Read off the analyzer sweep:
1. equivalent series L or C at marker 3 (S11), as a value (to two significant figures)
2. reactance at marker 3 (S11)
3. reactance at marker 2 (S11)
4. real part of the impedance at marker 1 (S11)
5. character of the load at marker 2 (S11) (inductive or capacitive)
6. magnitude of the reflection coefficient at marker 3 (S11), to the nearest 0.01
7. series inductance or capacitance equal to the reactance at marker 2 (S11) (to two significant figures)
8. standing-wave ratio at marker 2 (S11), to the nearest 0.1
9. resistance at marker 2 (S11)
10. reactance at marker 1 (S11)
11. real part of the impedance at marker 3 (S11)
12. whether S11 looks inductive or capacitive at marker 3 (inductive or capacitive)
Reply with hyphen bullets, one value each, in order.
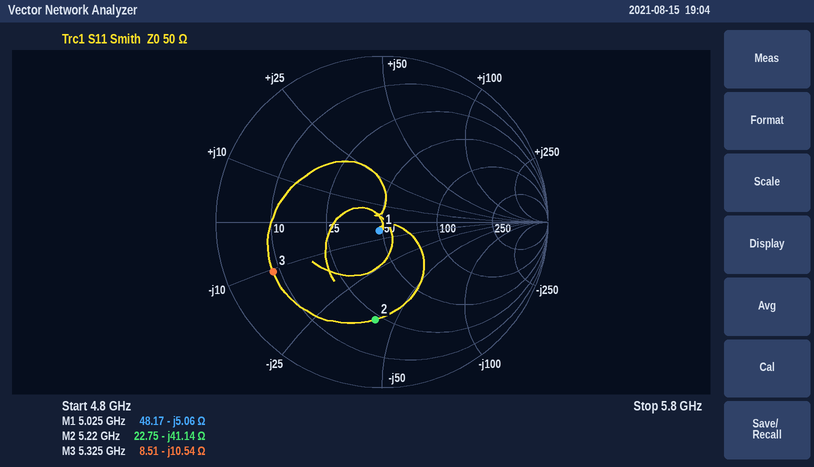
- 2.8 pF
- -10.54 Ω
- -41.14 Ω
- 48.17 Ω
- capacitive
- 0.72
- 740 fF
- 3.9
- 22.75 Ω
- -5.06 Ω
- 8.51 Ω
- capacitive
